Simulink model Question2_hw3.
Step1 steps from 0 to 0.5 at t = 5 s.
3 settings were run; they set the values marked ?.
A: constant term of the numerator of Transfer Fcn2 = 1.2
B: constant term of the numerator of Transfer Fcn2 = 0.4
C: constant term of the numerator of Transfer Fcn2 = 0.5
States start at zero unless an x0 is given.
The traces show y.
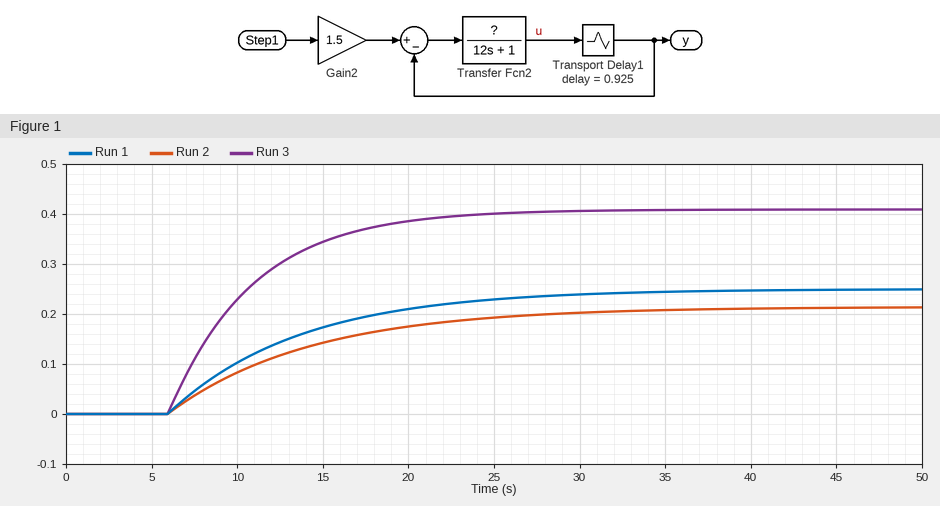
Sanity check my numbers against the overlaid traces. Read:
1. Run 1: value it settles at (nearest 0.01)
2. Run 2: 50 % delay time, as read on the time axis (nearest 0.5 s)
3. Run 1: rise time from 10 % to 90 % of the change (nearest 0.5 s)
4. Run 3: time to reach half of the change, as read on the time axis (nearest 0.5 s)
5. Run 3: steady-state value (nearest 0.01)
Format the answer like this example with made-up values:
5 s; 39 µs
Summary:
0.25; 11.5 s; 17.0 s; 9.5 s; 0.41
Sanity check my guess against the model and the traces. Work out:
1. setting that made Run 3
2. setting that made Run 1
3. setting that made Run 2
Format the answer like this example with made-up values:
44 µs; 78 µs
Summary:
A; C; B
